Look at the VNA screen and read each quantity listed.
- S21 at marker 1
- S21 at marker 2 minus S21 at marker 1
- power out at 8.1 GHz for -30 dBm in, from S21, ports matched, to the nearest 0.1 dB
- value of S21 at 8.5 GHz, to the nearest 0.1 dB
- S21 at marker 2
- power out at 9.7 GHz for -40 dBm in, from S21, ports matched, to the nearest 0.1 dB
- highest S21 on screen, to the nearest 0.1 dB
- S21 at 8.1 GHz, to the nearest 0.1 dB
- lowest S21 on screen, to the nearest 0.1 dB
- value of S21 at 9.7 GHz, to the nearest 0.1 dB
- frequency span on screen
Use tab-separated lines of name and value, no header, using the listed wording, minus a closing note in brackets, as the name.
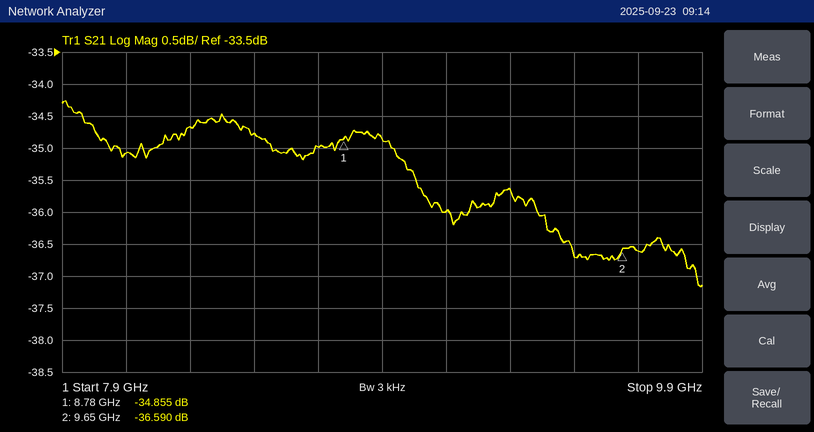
S21 at marker 1	-34.855 dB
S21 at marker 2 minus S21 at marker 1	-1.735 dB
power out at 8.1 GHz for -30 dBm in, from S21, ports matched, to the nearest 0.1 dB	-65.1 dBm
value of S21 at 8.5 GHz, to the nearest 0.1 dB	-34.8 dB
S21 at marker 2	-36.590 dB
power out at 9.7 GHz for -40 dBm in, from S21, ports matched, to the nearest 0.1 dB	-76.6 dBm
highest S21 on screen, to the nearest 0.1 dB	-34.3 dB
S21 at 8.1 GHz, to the nearest 0.1 dB	-35.1 dB
lowest S21 on screen, to the nearest 0.1 dB	-37.2 dB
value of S21 at 9.7 GHz, to the nearest 0.1 dB	-36.6 dB
frequency span on screen	2 GHz
